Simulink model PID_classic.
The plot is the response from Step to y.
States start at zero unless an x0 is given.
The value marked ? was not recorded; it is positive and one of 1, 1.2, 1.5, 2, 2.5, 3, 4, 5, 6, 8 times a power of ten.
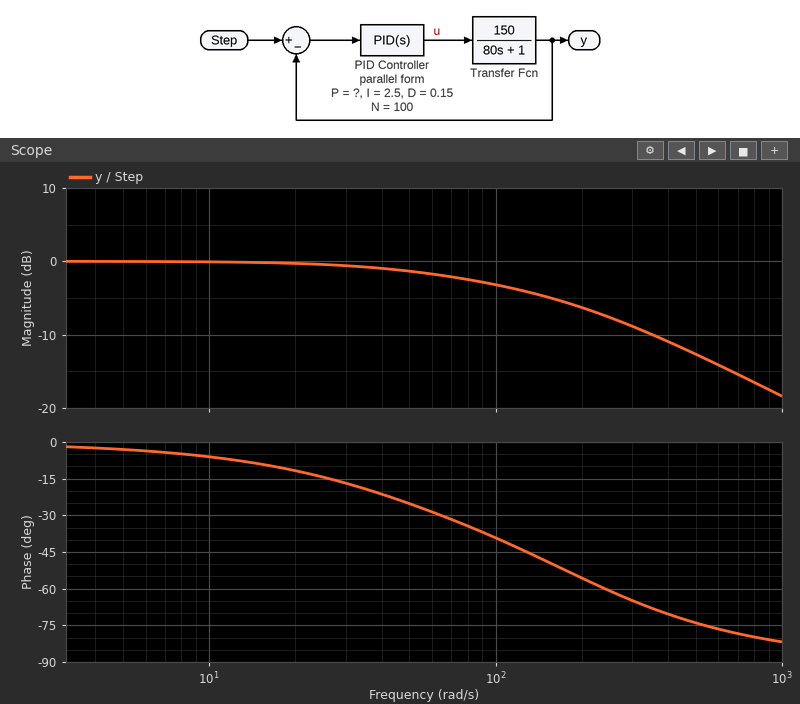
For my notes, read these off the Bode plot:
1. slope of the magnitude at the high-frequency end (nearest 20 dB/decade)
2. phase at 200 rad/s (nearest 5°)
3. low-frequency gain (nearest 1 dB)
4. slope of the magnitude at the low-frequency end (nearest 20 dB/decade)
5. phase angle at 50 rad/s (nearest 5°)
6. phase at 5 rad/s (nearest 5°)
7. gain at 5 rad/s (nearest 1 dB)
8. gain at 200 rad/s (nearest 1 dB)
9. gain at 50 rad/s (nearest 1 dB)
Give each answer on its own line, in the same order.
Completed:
-20 dB/decade
-55°
0 dB
0 dB/decade
-25°
-5°
0 dB
-6 dB
-1 dB
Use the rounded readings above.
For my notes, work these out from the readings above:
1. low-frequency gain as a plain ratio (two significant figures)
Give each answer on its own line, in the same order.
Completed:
1.0
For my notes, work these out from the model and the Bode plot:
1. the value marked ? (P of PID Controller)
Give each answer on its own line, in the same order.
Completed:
50
